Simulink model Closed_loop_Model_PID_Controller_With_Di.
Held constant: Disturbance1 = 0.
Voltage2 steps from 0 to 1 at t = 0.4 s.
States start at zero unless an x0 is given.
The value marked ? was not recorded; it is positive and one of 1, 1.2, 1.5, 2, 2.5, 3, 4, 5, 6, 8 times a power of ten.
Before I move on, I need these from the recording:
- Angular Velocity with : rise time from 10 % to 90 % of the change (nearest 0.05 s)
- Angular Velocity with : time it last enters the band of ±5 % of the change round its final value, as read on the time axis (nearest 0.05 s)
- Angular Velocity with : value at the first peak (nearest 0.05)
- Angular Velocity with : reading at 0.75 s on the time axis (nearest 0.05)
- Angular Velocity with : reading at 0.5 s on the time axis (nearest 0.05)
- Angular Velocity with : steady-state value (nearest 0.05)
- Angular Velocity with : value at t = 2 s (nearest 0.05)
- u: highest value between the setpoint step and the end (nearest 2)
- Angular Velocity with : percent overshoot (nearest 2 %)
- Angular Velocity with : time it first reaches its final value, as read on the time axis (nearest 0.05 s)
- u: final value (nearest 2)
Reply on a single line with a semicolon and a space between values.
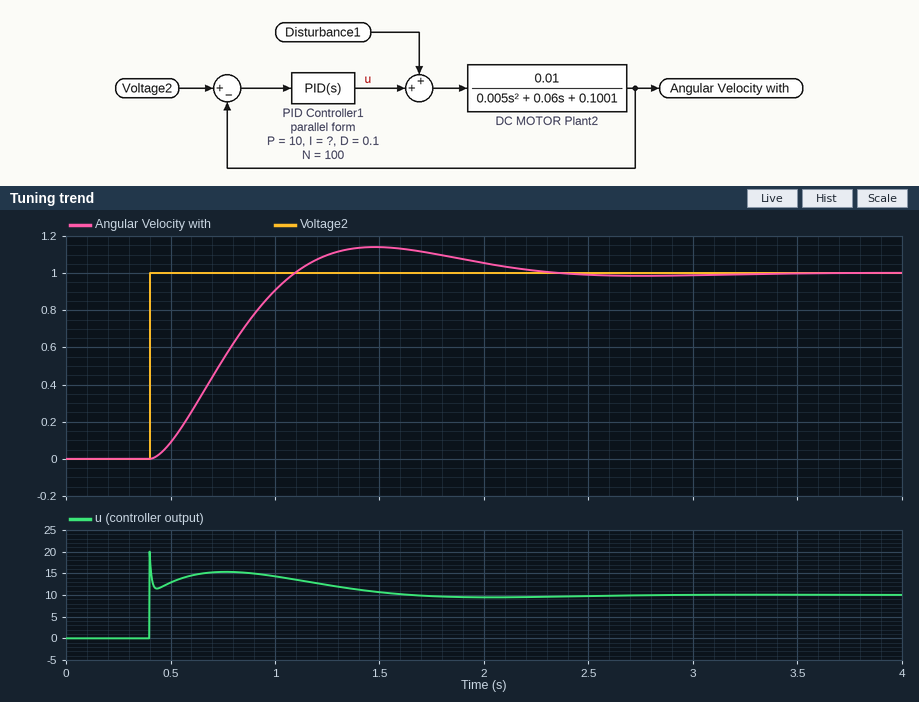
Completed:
0.50 s; 2.00 s; 1.15; 0.55; 0.10; 1.00; 1.05; 20; 14 %; 1.10 s; 10
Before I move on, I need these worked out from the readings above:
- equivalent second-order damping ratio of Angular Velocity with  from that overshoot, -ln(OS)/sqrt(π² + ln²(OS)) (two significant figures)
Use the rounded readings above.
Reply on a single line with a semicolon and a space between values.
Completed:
0.53
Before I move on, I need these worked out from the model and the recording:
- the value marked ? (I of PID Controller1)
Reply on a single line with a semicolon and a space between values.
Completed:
40
